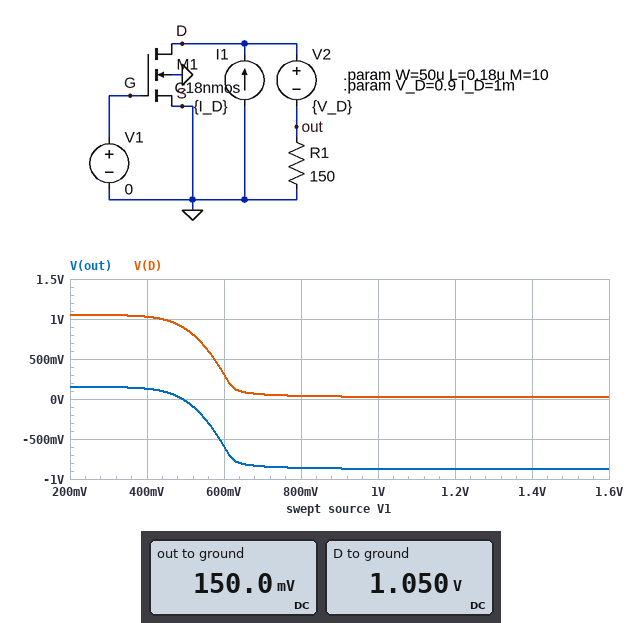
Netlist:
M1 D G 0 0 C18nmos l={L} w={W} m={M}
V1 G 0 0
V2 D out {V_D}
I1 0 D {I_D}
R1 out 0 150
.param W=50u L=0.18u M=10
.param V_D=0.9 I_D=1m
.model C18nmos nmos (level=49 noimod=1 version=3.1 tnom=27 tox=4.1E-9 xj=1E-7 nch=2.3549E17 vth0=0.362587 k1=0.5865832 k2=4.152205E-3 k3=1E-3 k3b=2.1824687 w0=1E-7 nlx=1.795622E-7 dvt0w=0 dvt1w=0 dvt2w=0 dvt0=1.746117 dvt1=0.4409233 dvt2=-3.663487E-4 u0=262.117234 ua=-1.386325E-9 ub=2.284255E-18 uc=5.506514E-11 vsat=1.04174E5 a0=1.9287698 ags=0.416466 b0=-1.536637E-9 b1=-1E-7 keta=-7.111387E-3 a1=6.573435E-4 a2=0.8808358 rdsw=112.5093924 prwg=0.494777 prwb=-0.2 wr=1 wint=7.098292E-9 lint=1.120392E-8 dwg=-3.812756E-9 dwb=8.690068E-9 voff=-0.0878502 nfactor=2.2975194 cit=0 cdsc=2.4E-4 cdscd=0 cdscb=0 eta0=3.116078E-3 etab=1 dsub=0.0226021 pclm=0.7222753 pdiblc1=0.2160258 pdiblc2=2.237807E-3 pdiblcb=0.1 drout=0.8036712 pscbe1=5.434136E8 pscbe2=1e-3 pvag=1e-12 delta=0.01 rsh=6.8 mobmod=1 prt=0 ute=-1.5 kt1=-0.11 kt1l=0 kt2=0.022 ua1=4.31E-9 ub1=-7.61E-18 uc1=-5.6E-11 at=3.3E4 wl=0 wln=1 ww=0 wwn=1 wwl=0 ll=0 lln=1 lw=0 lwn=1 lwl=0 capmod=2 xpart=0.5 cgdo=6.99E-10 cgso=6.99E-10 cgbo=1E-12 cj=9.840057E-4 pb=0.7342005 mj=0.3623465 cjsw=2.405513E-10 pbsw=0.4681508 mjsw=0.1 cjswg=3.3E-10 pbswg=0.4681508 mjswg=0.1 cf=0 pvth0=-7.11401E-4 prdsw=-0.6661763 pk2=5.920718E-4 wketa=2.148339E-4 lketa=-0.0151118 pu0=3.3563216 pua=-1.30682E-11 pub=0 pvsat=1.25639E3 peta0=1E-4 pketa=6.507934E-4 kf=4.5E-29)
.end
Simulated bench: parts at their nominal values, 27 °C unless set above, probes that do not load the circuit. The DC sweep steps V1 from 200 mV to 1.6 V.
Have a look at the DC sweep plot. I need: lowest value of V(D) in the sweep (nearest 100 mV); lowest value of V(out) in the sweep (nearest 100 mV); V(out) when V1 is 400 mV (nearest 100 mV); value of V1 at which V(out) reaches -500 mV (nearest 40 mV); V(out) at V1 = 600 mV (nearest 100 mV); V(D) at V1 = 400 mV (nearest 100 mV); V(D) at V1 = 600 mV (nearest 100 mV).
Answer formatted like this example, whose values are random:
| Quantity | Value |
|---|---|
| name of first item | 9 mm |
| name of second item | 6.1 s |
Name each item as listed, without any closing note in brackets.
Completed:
| Quantity | Value |
|---|---|
| lowest value of V(D) in the sweep | 0 V |
| lowest value of V(out) in the sweep | -900 mV |
| V(out) when V1 is 400 mV | 100 mV |
| value of V1 at which V(out) reaches -500 mV | 600 mV |
| V(out) at V1 = 600 mV | -600 mV |
| V(D) at V1 = 400 mV | 1.0 V |
| V(D) at V1 = 600 mV | 300 mV |
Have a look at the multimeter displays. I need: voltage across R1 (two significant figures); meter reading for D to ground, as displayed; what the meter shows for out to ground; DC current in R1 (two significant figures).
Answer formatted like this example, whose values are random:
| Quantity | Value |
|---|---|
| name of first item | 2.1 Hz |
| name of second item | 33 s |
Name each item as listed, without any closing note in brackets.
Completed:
| Quantity | Value |
|---|---|
| voltage across R1 | 150 mV |
| meter reading for D to ground, as displayed | 1.050 V |
| what the meter shows for out to ground | 150.0 mV |
| DC current in R1 | 1.0 mA |
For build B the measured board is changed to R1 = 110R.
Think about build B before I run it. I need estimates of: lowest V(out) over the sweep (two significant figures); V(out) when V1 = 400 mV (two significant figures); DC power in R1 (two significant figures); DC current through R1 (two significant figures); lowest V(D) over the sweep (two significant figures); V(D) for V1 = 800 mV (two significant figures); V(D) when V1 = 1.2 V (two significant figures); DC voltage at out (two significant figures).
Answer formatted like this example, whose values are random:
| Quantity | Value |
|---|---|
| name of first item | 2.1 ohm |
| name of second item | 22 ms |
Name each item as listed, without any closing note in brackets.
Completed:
| Quantity | Value |
|---|---|
| lowest V(out) over the sweep | -870 mV |
| V(out) when V1 = 400 mV | 95 mV |
| DC power in R1 | 110 µW |
| DC current through R1 | 1.0 mA |
| lowest V(D) over the sweep | 26 mV |
| V(D) for V1 = 800 mV | 52 mV |
| V(D) when V1 = 1.2 V | 30 mV |
| DC voltage at out | 110 mV |
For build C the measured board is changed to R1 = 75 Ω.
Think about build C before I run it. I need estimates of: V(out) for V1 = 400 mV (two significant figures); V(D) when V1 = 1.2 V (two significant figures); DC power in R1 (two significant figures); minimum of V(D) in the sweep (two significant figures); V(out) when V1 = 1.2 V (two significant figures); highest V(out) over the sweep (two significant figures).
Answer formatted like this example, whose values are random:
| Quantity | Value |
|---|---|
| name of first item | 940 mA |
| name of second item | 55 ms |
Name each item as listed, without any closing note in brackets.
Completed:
| Quantity | Value |
|---|---|
| V(out) for V1 = 400 mV | 65 mV |
| V(D) when V1 = 1.2 V | 43 mV |
| DC power in R1 | 75 µW |
| minimum of V(D) in the sweep | 36 mV |
| V(out) when V1 = 1.2 V | -860 mV |
| highest V(out) over the sweep | 75 mV |
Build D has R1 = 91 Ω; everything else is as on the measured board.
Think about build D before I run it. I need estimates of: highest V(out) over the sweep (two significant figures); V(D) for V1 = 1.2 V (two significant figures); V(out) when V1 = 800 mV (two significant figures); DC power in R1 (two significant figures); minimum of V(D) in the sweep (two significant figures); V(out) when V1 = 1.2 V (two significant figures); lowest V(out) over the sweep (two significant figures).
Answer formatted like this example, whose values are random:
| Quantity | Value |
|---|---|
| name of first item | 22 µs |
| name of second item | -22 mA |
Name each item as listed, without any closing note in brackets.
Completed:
| Quantity | Value |
|---|---|
| highest V(out) over the sweep | 91 mV |
| V(D) for V1 = 1.2 V | 36 mV |
| V(out) when V1 = 800 mV | -840 mV |
| DC power in R1 | 91 µW |
| minimum of V(D) in the sweep | 31 mV |
| V(out) when V1 = 1.2 V | -860 mV |
| lowest V(out) over the sweep | -870 mV |
